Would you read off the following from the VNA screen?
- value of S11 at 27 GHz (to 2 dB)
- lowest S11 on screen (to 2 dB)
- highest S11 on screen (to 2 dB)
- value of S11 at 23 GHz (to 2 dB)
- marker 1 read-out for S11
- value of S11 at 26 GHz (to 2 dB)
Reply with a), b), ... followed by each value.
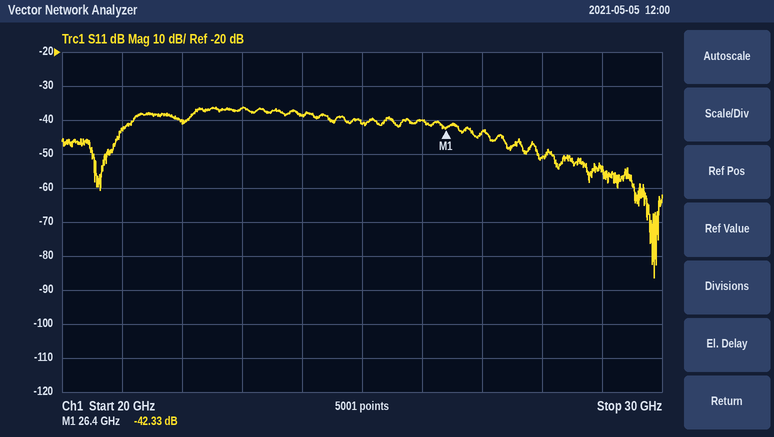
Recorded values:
a) -44 dB
b) -86 dB
c) -36 dB
d) -36 dB
e) -42.33 dB
f) -40 dB
